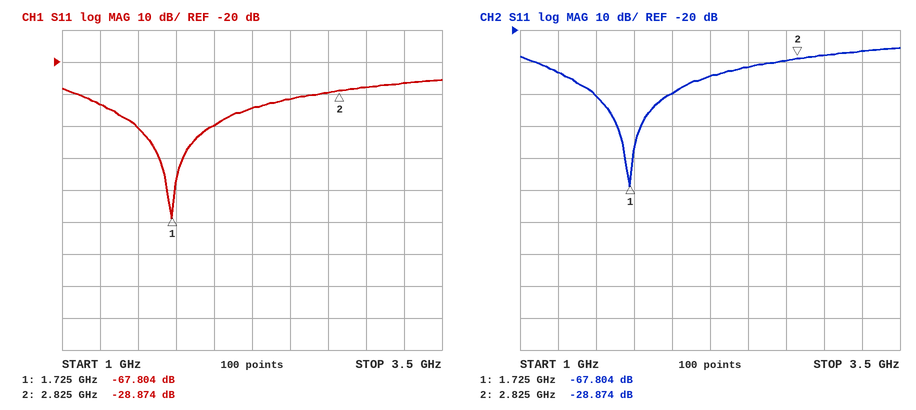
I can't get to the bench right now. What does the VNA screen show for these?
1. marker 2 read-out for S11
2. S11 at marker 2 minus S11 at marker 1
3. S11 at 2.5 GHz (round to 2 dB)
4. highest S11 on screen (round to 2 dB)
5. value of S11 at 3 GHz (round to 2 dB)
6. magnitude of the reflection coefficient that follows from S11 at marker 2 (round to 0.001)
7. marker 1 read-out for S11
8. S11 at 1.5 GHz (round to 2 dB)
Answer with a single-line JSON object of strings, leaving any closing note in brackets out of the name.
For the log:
{"marker 2 read-out for S11": "-28.874 dB", "S11 at marker 2 minus S11 at marker 1": "38.930 dB", "S11 at 2.5 GHz": "-32 dB", "highest S11 on screen": "-26 dB", "value of S11 at 3 GHz": "-28 dB", "magnitude of the reflection coefficient that follows from S11 at marker 2": "0.036", "marker 1 read-out for S11": "-67.804 dB", "S11 at 1.5 GHz": "-40 dB"}
